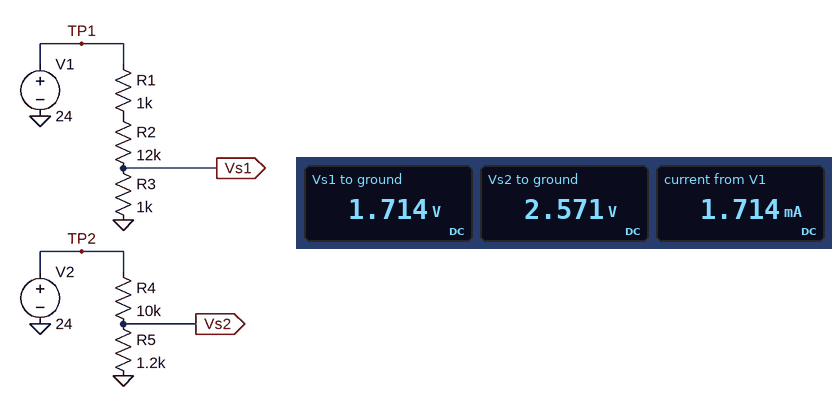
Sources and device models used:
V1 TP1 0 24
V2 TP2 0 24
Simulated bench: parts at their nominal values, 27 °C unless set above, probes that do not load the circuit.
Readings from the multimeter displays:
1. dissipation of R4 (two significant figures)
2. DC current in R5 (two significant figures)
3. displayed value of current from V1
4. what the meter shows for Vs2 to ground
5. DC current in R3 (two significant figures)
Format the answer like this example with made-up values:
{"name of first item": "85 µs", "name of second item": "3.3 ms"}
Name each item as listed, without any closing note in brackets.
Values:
{"dissipation of R4": "46 mW", "DC current in R5": "2.1 mA", "displayed value of current from V1": "1.714 mA", "what the meter shows for Vs2 to ground": "2.571 V", "DC current in R3": "1.7 mA"}
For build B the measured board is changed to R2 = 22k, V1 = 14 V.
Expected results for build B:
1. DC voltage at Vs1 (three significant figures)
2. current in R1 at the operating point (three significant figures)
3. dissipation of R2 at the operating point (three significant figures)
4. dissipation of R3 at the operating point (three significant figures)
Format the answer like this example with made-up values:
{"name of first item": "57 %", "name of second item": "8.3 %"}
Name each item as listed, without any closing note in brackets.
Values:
{"DC voltage at Vs1": "583 mV", "current in R1 at the operating point": "583 µA", "dissipation of R2 at the operating point": "7.49 mW", "dissipation of R3 at the operating point": "340 µW"}
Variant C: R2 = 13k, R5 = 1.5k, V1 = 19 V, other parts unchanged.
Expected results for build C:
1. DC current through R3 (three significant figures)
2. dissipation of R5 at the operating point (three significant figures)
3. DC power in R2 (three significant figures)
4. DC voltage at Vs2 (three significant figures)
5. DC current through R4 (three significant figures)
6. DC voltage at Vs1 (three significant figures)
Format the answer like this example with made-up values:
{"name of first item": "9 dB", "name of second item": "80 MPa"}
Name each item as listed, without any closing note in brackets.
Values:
{"DC current through R3": "1.27 mA", "dissipation of R5 at the operating point": "6.53 mW", "DC power in R2": "20.9 mW", "DC voltage at Vs2": "3.13 V", "DC current through R4": "2.09 mA", "DC voltage at Vs1": "1.27 V"}
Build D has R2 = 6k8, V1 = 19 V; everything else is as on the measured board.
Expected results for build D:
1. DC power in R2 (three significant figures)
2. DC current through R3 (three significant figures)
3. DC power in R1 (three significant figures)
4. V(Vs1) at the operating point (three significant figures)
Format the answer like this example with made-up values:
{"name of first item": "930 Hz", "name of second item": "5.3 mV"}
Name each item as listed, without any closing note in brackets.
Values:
{"DC power in R2": "31.7 mW", "DC current through R3": "2.16 mA", "DC power in R1": "4.66 mW", "V(Vs1) at the operating point": "2.16 V"}
